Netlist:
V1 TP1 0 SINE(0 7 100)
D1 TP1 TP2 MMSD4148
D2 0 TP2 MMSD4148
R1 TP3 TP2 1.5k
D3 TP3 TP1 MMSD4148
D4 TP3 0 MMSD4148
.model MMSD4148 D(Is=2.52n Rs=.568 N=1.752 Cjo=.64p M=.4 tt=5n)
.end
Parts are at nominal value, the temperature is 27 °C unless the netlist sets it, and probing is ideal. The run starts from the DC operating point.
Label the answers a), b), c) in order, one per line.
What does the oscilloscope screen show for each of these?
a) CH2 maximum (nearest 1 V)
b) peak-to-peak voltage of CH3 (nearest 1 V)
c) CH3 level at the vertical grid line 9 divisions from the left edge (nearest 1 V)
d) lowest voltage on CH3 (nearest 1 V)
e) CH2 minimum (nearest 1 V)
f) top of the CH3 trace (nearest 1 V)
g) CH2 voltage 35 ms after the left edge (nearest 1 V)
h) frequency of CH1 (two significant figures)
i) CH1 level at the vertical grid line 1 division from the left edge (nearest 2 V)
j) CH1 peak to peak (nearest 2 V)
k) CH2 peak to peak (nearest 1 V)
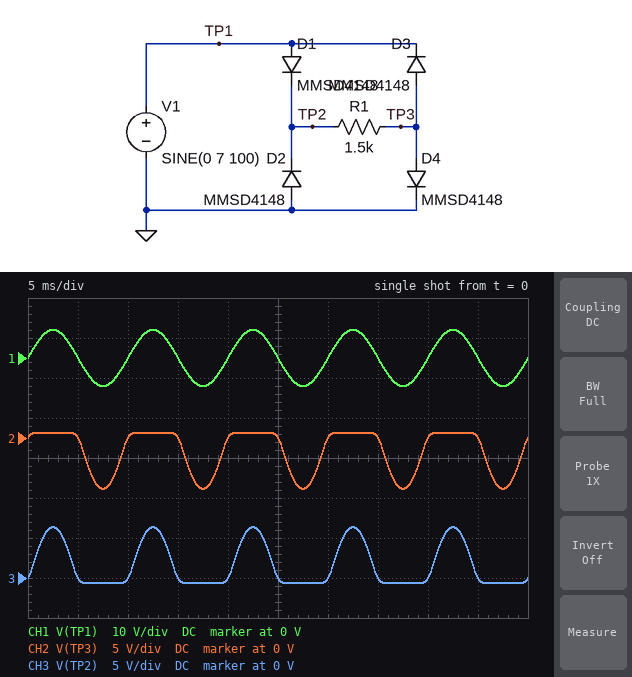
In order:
a) 1 V
b) 7 V
c) 0 V
d) -1 V
e) -6 V
f) 6 V
g) 0 V
h) 100 Hz
i) 0 V
j) 14 V
k) 7 V
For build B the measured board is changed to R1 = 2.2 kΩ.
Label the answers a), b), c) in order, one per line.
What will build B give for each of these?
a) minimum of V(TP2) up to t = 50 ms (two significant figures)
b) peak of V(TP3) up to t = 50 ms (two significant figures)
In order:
a) -630 mV
b) 630 mV
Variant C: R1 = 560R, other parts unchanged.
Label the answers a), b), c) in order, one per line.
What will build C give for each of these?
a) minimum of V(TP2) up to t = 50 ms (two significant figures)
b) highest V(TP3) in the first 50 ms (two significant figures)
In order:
a) -690 mV
b) 690 mV
